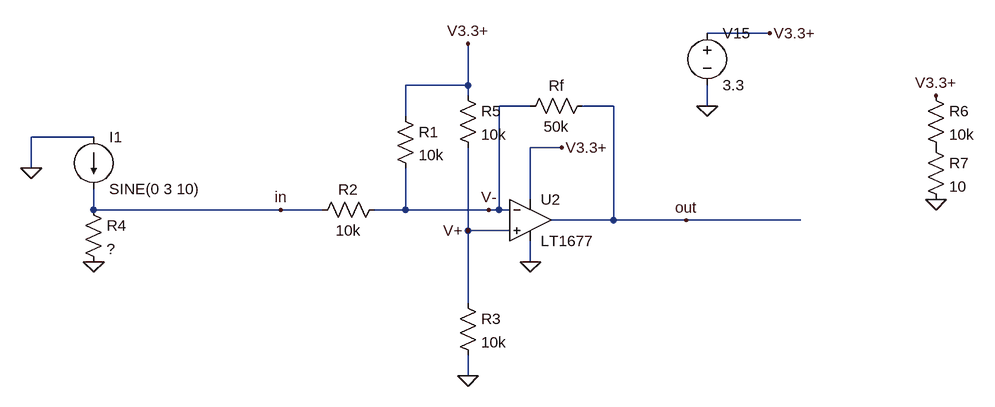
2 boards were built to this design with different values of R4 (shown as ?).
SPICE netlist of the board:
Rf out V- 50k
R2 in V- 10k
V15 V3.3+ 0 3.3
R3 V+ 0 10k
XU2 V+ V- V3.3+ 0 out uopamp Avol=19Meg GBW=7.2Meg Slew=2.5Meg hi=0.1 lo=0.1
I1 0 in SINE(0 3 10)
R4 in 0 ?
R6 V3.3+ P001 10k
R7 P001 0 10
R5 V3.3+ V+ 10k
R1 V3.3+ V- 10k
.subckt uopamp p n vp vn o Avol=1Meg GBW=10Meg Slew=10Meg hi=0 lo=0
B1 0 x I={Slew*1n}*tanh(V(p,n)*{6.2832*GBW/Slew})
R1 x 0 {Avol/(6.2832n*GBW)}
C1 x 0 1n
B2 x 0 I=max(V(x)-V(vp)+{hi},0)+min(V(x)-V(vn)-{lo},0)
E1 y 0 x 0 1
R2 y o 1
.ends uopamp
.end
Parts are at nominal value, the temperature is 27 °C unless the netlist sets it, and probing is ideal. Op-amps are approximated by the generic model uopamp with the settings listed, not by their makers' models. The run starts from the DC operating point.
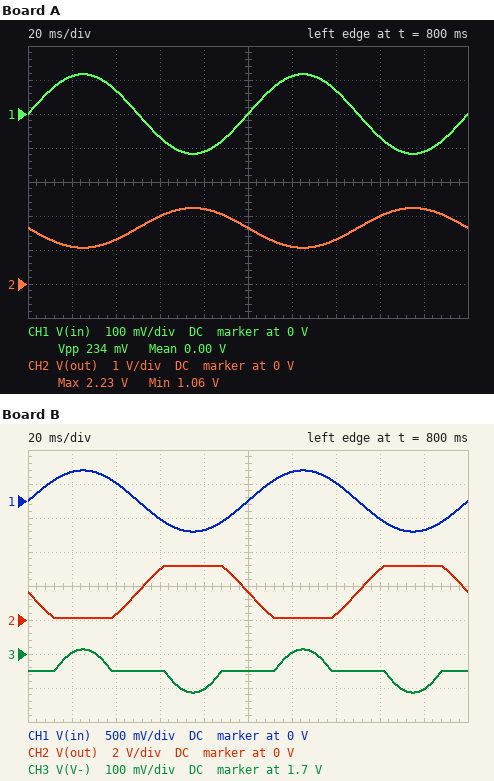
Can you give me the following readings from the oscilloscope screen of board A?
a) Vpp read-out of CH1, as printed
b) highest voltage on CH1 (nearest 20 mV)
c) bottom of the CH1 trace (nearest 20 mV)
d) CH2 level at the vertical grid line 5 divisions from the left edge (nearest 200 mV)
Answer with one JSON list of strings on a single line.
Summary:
["234 mV", "120 mV", "-120 mV", "1.6 V"]
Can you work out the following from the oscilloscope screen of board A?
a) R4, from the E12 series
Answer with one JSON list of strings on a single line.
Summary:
["0.039 Ω"]
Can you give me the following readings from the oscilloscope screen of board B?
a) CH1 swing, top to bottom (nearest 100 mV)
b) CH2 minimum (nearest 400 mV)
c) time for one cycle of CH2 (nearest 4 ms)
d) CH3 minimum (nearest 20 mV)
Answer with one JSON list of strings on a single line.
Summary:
["900 mV", "0 V", "100 ms", "1.58 V"]
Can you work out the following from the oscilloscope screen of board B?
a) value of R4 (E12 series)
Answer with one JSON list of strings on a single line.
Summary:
["0.15 Ω"]
